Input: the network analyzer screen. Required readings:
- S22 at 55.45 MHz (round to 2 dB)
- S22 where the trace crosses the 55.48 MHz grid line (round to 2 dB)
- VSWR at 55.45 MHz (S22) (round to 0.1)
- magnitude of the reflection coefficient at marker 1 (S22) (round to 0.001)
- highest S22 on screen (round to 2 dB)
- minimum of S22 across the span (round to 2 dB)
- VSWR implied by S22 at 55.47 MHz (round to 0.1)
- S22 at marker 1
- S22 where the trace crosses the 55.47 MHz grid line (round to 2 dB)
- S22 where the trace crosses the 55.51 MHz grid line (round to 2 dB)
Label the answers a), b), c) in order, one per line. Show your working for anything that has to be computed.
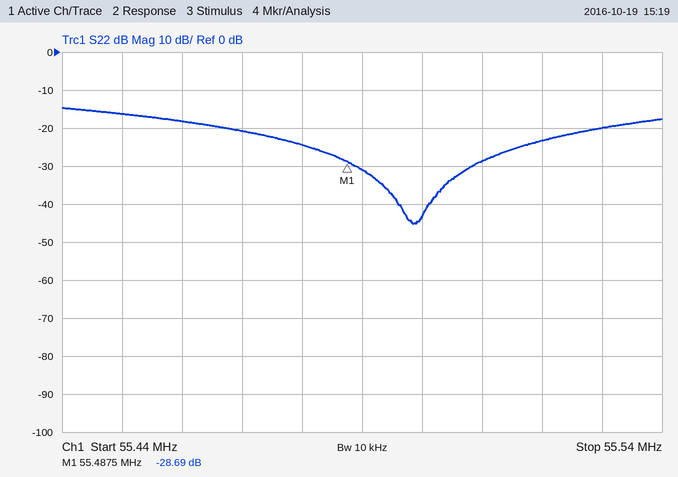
a) -16 dB
b) -24 dB
c) |Γ| = 10^(-16/20) = 0.1585; VSWR = (1 + 0.1585)/(1 − 0.1585) ≈ 1.4
d) 10^(-28.69/20) ≈ 0.037
e) -14 dB
f) -46 dB
g) |Γ| = 10^(-20/20) = 0.1000; VSWR = (1 + 0.1000)/(1 − 0.1000) ≈ 1.2
h) -28.69 dB
i) -20 dB
j) -28 dB
